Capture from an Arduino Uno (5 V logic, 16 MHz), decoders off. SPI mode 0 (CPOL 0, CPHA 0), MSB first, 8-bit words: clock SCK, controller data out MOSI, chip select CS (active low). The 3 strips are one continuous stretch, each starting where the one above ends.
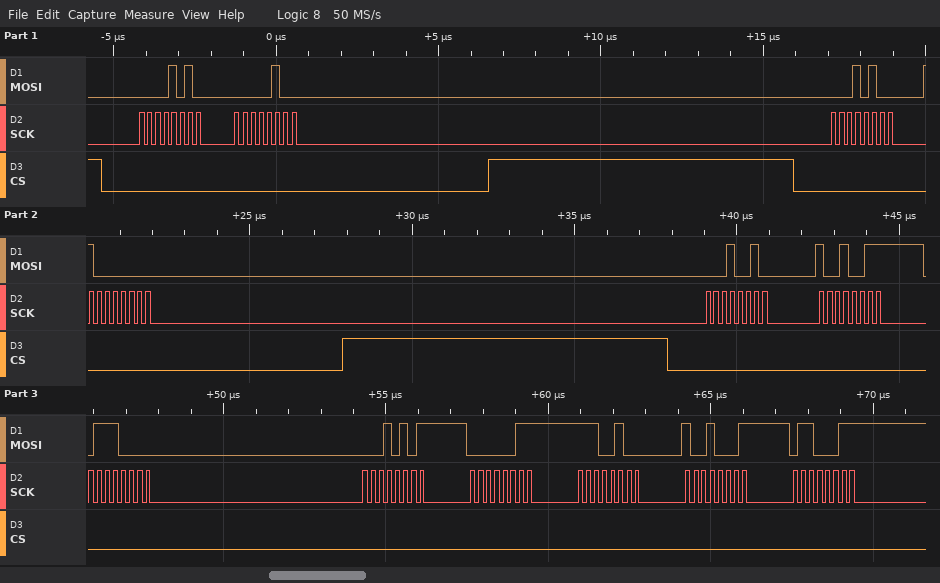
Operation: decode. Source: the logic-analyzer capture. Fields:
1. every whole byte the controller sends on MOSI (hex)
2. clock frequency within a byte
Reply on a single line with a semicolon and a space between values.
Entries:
0A 04 14 80 12 93 70 15 03 E4 91 63; 4 MHz
